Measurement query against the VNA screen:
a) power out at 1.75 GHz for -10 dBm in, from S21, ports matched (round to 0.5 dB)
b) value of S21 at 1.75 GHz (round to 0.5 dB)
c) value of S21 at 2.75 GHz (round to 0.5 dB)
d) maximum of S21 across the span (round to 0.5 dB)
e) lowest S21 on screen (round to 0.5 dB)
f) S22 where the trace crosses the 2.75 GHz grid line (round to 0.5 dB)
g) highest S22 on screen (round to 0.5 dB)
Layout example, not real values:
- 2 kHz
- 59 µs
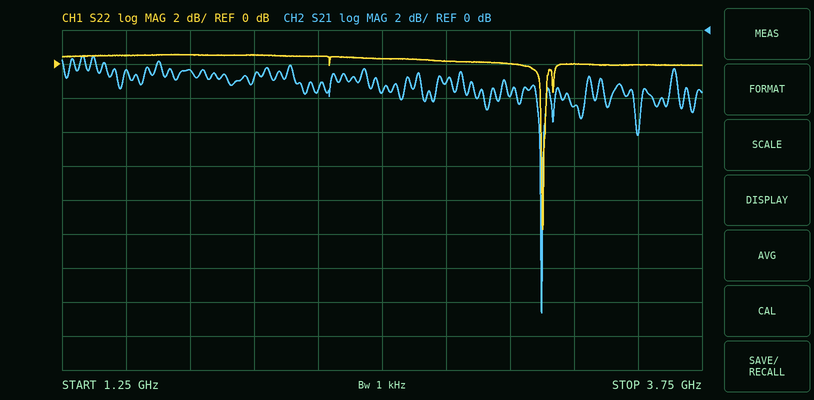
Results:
- -12.5 dBm
- -2.5 dB
- -3.0 dB
- -1.5 dB
- -16.5 dB
- 0.0 dB
- 0.5 dB
